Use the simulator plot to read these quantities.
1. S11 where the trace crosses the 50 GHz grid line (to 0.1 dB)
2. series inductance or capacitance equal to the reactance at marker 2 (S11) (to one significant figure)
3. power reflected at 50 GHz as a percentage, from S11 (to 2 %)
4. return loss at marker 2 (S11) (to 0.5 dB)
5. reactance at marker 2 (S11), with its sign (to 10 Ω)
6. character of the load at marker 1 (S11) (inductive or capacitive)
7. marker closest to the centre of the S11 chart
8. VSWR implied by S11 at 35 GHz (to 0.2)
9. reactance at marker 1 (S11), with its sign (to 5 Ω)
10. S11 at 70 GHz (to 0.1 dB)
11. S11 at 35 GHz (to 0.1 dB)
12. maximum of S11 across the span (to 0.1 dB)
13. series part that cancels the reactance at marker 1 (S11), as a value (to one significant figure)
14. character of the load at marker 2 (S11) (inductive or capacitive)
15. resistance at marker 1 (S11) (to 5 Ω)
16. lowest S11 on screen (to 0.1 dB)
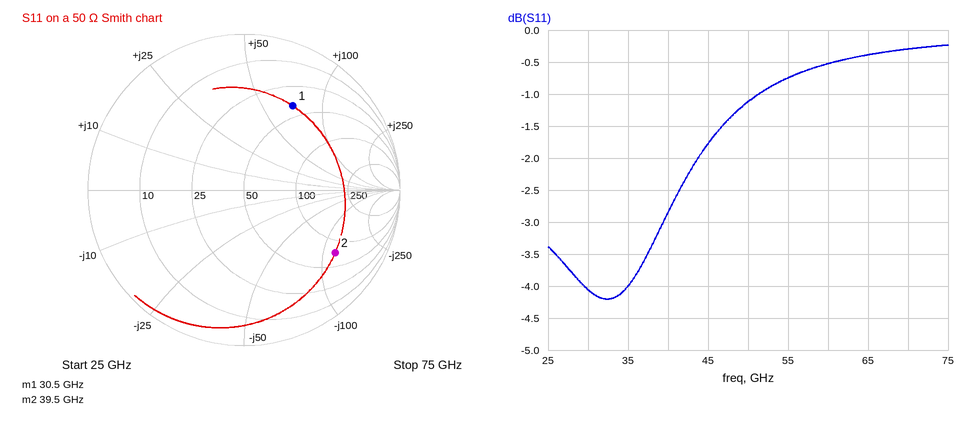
-1.1 dB
30 fF
78 %
3.0 dB
-120 Ω
inductive
marker 1
4.4
+70 Ω
-0.3 dB
-4.0 dB
-0.2 dB
70 fF
capacitive
40 Ω
-4.2 dB
